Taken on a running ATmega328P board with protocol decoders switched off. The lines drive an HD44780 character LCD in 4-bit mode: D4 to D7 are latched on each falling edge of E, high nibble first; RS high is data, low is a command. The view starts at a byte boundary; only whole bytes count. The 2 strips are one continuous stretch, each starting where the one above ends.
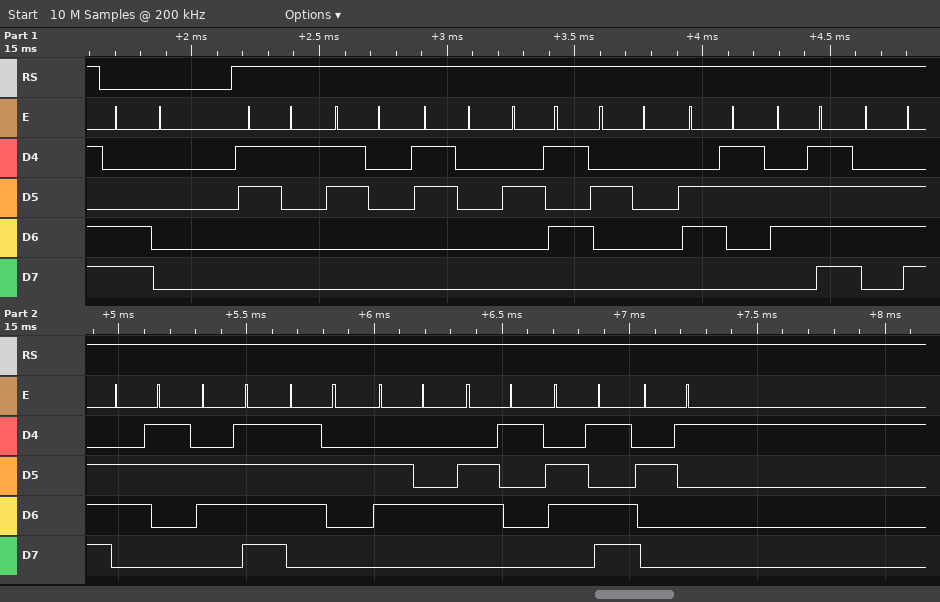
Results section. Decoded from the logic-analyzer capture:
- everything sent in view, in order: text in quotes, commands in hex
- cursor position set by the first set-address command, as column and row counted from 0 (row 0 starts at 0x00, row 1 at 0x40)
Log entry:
0xC0 "100% concordam!"
column 0, row 1
